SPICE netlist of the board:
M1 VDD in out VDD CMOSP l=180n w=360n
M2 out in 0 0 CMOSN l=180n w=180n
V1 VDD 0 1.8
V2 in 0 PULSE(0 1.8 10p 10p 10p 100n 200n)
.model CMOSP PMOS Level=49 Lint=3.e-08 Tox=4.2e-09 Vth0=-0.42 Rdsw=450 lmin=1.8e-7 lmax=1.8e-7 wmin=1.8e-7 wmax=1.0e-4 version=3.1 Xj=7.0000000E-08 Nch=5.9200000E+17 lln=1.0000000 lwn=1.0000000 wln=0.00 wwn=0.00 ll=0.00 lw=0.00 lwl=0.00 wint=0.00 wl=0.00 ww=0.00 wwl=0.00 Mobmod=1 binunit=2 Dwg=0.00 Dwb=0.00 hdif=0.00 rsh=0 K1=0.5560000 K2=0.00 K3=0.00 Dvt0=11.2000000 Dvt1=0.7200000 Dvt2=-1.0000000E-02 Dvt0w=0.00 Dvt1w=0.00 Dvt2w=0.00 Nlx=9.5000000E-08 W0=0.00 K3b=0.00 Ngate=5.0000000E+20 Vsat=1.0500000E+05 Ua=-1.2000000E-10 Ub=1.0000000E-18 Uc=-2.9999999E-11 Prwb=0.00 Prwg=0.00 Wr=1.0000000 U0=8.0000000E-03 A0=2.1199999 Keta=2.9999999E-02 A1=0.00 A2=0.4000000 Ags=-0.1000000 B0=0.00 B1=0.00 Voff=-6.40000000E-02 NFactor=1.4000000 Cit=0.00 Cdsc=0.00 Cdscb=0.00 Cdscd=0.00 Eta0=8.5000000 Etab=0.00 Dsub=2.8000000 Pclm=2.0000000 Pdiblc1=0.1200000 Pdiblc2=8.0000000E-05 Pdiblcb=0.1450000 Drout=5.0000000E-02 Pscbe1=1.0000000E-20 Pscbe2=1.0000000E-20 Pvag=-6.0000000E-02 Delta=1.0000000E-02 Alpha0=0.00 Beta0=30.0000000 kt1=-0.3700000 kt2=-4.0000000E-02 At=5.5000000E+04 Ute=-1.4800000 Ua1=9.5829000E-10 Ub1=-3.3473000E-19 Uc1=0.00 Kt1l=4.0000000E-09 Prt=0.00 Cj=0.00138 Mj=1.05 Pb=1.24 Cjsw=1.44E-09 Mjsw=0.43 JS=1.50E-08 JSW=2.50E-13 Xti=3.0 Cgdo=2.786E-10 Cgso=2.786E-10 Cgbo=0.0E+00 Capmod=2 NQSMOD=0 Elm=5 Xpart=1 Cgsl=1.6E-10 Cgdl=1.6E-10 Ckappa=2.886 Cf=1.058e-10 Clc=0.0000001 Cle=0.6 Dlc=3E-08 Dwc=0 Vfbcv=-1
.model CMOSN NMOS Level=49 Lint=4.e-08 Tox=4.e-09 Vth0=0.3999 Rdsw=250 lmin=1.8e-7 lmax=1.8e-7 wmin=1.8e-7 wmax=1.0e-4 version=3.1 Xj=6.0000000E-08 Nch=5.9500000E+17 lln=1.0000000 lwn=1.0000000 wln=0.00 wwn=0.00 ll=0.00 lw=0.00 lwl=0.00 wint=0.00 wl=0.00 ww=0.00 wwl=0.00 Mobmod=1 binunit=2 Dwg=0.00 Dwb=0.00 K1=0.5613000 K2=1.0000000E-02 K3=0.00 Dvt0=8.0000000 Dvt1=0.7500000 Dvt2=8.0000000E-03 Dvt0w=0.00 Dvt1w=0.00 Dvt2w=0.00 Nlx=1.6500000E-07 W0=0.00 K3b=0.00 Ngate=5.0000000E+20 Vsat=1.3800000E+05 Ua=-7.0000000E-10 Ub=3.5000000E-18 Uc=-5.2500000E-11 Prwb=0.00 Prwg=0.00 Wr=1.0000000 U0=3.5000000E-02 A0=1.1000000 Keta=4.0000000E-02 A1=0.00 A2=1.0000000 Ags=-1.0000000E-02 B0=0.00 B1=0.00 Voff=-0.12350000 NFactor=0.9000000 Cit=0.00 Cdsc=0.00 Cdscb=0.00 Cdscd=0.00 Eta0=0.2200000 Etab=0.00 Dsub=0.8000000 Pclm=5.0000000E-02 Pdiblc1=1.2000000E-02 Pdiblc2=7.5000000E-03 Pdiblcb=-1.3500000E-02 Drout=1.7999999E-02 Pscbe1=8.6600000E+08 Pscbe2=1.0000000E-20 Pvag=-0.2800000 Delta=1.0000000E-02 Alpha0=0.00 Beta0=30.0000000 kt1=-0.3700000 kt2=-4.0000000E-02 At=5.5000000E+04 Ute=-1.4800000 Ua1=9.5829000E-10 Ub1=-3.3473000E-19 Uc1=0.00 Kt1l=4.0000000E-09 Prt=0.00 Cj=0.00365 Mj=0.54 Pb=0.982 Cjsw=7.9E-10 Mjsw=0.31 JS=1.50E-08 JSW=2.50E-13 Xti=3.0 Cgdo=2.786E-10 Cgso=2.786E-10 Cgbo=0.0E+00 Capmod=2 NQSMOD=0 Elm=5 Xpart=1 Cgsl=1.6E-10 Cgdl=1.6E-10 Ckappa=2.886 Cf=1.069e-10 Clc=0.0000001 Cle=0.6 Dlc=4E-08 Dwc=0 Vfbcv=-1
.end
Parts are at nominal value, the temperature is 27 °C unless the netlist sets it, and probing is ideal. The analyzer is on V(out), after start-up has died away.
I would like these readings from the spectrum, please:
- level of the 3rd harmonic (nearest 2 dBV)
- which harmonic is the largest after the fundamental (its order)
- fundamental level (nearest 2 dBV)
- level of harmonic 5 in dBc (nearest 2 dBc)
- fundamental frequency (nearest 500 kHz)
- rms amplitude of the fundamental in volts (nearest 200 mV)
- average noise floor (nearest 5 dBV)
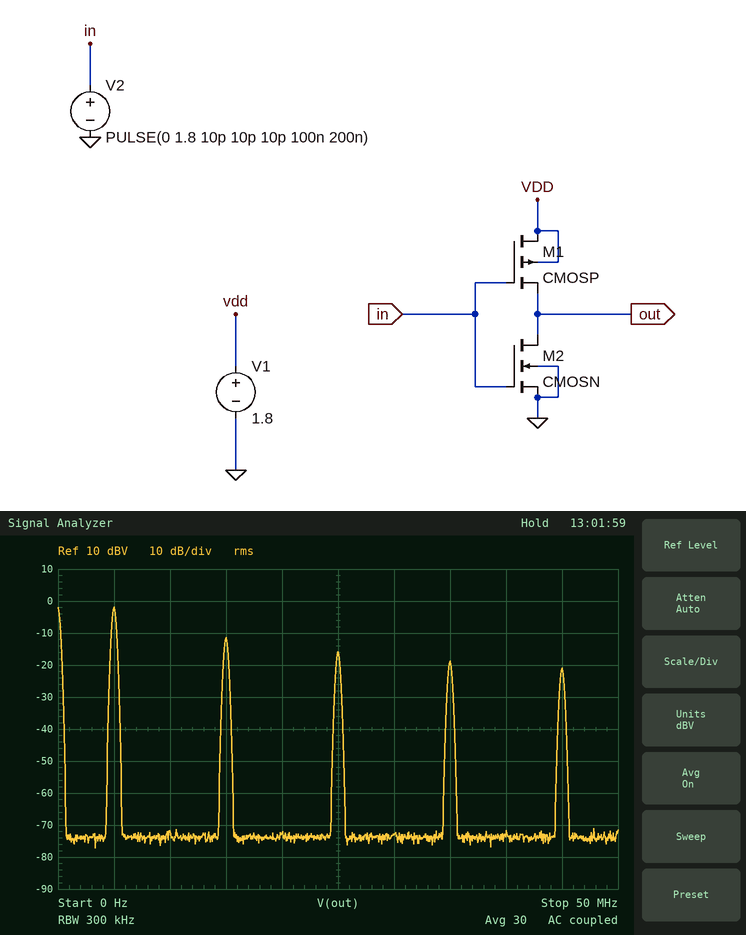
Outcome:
-12 dBV
3
-2 dBV
-14 dBc
5.0 MHz
800 mV
-75 dBV
